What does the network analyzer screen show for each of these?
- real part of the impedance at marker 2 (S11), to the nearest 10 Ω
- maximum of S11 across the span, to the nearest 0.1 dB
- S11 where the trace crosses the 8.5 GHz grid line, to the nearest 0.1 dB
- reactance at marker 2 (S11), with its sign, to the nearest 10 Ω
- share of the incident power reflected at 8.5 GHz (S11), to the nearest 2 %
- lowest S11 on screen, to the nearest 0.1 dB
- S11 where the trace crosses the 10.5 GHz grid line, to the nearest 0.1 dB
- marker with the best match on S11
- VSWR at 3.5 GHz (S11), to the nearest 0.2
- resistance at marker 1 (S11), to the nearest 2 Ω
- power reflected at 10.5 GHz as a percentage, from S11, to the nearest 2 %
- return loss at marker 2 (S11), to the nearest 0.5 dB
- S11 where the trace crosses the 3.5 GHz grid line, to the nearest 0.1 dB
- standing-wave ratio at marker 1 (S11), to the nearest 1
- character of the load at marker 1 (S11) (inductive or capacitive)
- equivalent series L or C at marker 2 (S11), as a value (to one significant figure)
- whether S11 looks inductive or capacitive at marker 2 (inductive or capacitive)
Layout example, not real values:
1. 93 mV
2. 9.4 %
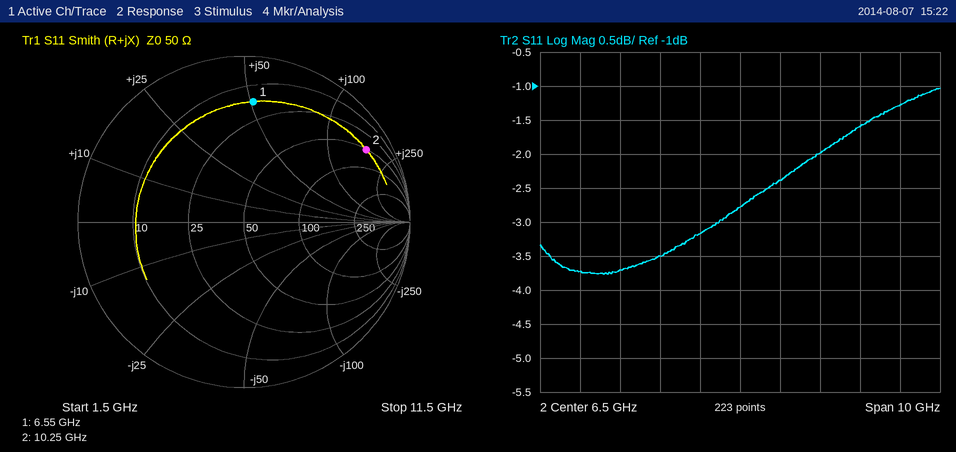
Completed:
1. 50 Ω
2. -1.0 dB
3. -2.0 dB
4. +170 Ω
5. 64 %
6. -3.8 dB
7. -1.3 dB
8. marker 1
9. 4.8
10. 16 Ω
11. 74 %
12. 1.5 dB
13. -3.7 dB
14. 6
15. inductive
16. 3 nH
17. inductive
